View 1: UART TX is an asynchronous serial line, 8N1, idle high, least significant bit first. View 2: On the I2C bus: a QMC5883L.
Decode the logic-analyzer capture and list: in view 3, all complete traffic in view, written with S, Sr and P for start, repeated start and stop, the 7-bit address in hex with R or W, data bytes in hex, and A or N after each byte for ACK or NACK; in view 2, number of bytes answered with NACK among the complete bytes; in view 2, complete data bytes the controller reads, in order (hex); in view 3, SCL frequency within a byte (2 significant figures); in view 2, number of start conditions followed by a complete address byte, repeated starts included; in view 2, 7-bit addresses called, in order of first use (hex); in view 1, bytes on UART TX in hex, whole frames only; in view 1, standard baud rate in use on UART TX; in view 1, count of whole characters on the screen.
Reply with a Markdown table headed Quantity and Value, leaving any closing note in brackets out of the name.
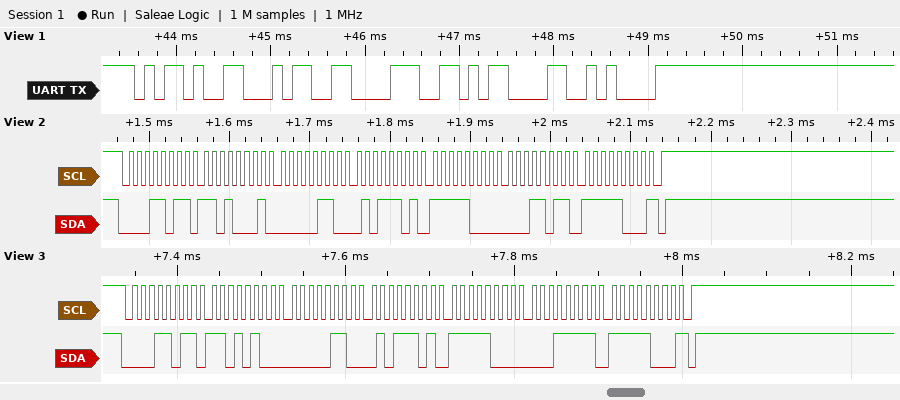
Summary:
| Quantity | Value |
|---|---|
| in view 3, all complete traffic in view, written with S, Sr and P for start, repeated start and stop, the 7-bit address in hex with R or W, data bytes in hex, and A or N after each byte for ACK or NACK | S 0DR A D4 A 06 A 5D A F8 A 1F A F8 N P |
| in view 2, number of bytes answered with NACK among the complete bytes | 1 |
| in view 2, complete data bytes the controller reads, in order | D1 06 5D F8 1B F8 |
| in view 3, SCL frequency within a byte | 100 kHz |
| in view 2, number of start conditions followed by a complete address byte, repeated starts included | 1 |
| in view 2, 7-bit addresses called, in order of first use | 0x0D |
| in view 1, bytes on UART TX in hex, whole frames only | 2D 34 38 0D 0A |
| in view 1, standard baud rate in use on UART TX | 9600 baud |
| in view 1, count of whole characters on the screen | 5 |
